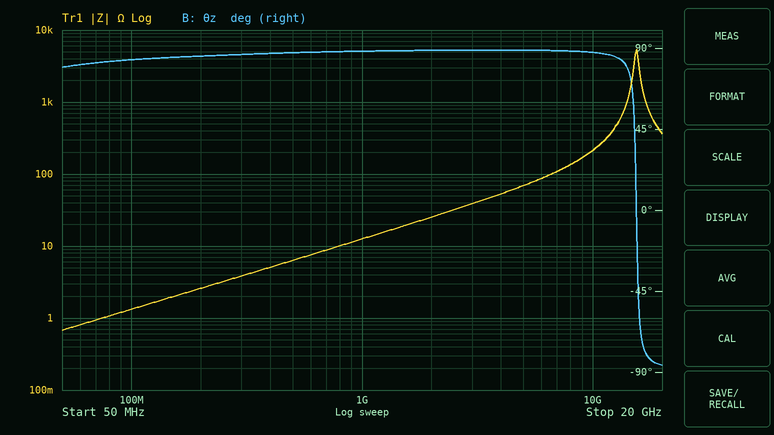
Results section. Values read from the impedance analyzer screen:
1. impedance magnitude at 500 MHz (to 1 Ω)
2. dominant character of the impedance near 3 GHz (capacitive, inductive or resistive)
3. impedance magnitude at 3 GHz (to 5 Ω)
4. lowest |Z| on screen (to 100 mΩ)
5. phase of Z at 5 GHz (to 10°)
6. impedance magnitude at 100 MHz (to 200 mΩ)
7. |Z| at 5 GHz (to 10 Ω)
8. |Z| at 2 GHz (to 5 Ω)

6 Ω
inductive
40 Ω
700 mΩ
90°
1.4 Ω
70 Ω
25 Ω
